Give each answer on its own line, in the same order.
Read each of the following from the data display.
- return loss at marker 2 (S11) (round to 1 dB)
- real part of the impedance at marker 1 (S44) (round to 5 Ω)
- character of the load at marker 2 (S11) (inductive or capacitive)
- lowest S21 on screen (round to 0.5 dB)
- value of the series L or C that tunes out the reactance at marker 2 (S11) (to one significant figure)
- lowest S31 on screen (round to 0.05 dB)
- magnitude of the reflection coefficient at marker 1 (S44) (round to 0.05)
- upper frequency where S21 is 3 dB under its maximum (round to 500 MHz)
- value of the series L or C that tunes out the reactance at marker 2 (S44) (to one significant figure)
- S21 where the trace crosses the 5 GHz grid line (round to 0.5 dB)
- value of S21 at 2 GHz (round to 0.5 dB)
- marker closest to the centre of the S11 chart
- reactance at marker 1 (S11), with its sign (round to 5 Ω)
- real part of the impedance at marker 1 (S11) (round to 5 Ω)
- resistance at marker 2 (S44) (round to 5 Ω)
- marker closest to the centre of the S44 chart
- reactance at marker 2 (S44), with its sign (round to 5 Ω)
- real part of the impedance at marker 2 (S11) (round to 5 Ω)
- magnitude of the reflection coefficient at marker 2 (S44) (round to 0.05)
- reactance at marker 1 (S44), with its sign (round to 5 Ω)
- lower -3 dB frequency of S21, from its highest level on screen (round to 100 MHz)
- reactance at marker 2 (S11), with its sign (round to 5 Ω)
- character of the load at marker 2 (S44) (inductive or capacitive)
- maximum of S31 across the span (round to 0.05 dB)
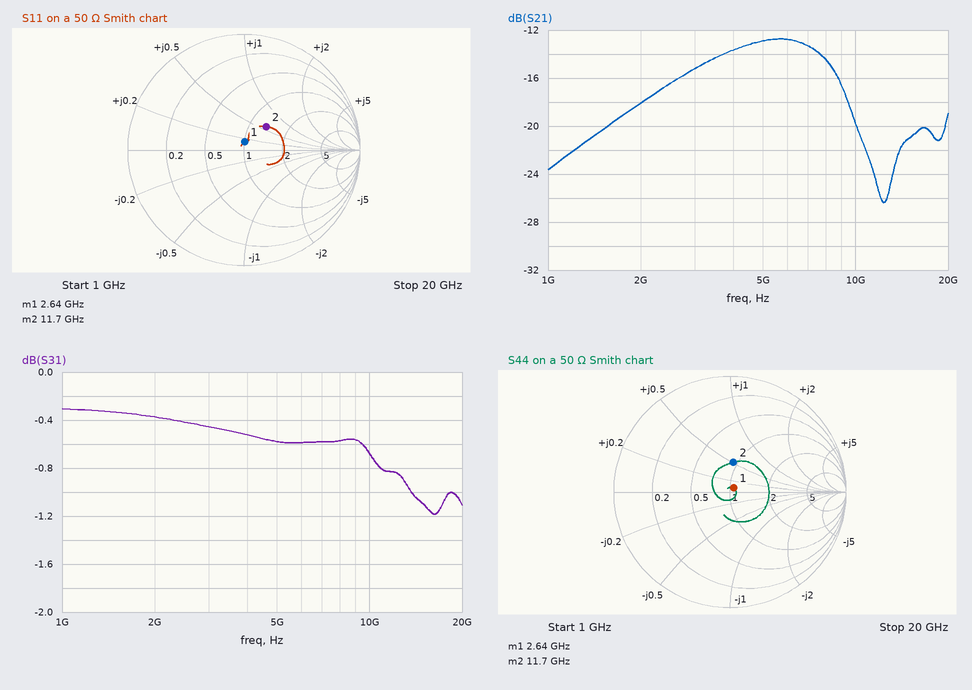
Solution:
11 dB
55 Ω
inductive
-26.5 dB
500 fF
-1.20 dB
0.05
8.5 GHz
500 fF
-13.0 dB
-18.0 dB
marker 1
+5 Ω
50 Ω
45 Ω
marker 1
+25 Ω
65 Ω
0.25
+5 Ω
2.8 GHz
+30 Ω
inductive
-0.30 dB
